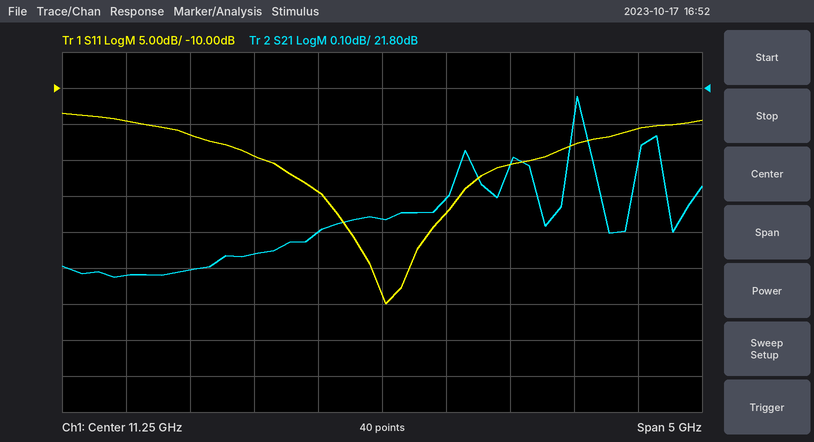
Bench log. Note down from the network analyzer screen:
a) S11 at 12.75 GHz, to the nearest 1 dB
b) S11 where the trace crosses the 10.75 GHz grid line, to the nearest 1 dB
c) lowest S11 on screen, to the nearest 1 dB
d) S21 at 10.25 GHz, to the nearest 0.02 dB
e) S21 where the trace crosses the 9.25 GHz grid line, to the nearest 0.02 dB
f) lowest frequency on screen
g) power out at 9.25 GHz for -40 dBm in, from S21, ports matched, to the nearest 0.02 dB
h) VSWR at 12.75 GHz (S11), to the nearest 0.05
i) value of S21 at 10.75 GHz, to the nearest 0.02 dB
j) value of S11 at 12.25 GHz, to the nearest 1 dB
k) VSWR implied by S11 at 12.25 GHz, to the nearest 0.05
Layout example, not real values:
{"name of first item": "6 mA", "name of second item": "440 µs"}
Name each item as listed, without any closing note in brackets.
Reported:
{"S11 at 12.75 GHz, to the nearest 1 dB": "-18 dB", "S11 where the trace crosses the 10.75 GHz grid line, to the nearest 1 dB": "-24 dB", "lowest S11 on screen, to the nearest 1 dB": "-40 dB", "S21 at 10.25 GHz, to the nearest 0.02 dB": "21.34 dB", "S21 where the trace crosses the 9.25 GHz grid line, to the nearest 0.02 dB": "21.28 dB", "lowest frequency on screen": "8.75 GHz", "power out at 9.25 GHz for -40 dBm in, from S21, ports matched, to the nearest 0.02 dB": "-18.72 dBm", "VSWR at 12.75 GHz (S11), to the nearest 0.05": "1.30", "value of S21 at 10.75 GHz, to the nearest 0.02 dB": "21.40 dB", "value of S11 at 12.25 GHz, to the nearest 1 dB": "-21 dB", "VSWR implied by S11 at 12.25 GHz, to the nearest 0.05": "1.20"}
